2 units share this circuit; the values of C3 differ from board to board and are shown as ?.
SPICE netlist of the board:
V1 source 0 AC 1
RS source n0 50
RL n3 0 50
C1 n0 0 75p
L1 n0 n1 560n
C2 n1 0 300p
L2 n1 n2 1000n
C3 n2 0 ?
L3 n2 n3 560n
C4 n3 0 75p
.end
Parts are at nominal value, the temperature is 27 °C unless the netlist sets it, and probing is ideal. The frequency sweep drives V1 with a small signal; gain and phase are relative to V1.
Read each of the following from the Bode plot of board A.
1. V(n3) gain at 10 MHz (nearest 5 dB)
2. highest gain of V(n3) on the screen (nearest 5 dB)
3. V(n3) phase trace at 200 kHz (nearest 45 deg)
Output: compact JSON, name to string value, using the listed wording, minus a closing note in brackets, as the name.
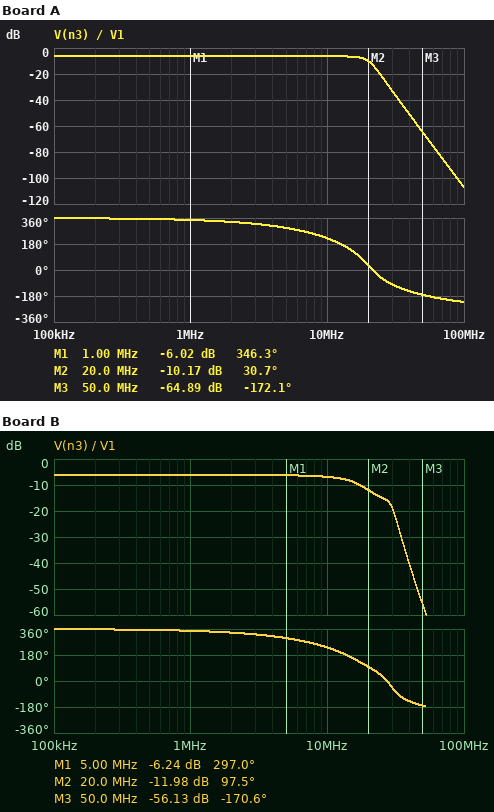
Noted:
{"V(n3) gain at 10 MHz": "-5 dB", "highest gain of V(n3) on the screen": "-5 dB", "V(n3) phase trace at 200 kHz": "360 deg"}
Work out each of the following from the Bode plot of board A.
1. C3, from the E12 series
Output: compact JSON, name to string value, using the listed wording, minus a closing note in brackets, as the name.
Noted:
{"C3, from the E12 series": "220 pF"}
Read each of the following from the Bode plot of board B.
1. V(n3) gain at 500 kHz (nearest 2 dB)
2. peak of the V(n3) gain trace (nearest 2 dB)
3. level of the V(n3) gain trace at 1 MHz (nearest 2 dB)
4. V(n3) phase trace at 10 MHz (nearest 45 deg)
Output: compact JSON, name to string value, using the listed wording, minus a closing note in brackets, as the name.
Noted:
{"V(n3) gain at 500 kHz": "-6 dB", "peak of the V(n3) gain trace": "-6 dB", "level of the V(n3) gain trace at 1 MHz": "-6 dB", "V(n3) phase trace at 10 MHz": "225 deg"}
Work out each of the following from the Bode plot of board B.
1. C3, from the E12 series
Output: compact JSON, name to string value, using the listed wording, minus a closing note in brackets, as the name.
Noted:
{"C3, from the E12 series": "100 pF"}
